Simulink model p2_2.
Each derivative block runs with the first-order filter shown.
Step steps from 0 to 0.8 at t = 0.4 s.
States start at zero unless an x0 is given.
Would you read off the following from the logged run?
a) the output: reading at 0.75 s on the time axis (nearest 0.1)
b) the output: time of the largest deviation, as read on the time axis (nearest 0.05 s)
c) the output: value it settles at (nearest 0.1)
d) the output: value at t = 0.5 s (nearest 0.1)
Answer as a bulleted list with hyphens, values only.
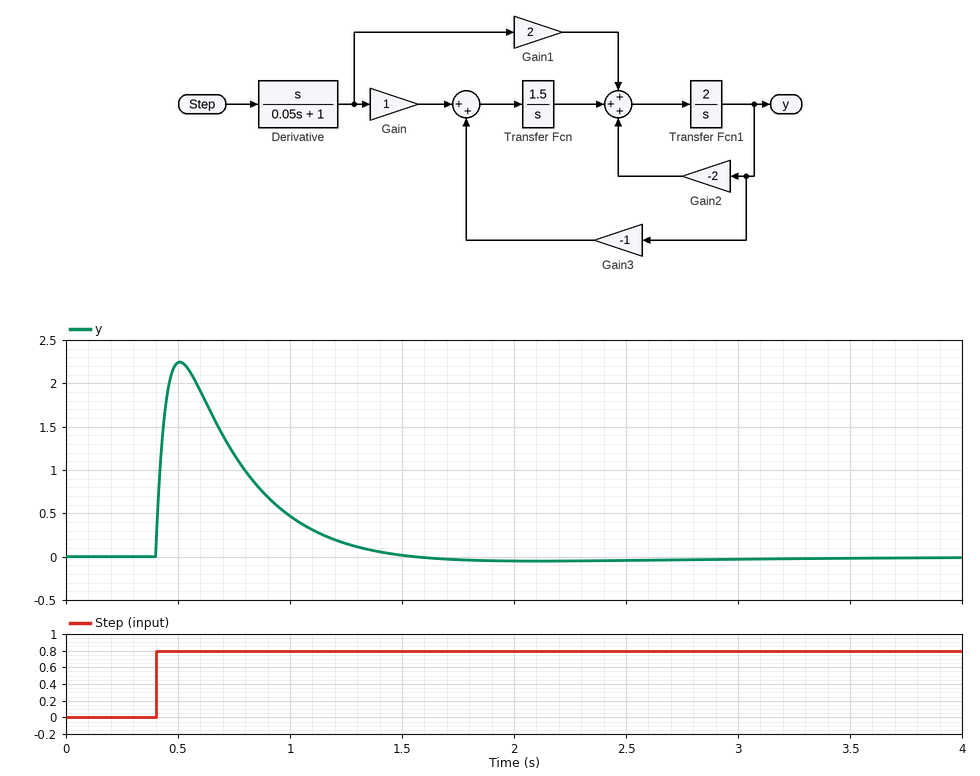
- 1.2
- 0.50 s
- 0.0
- 2.2
